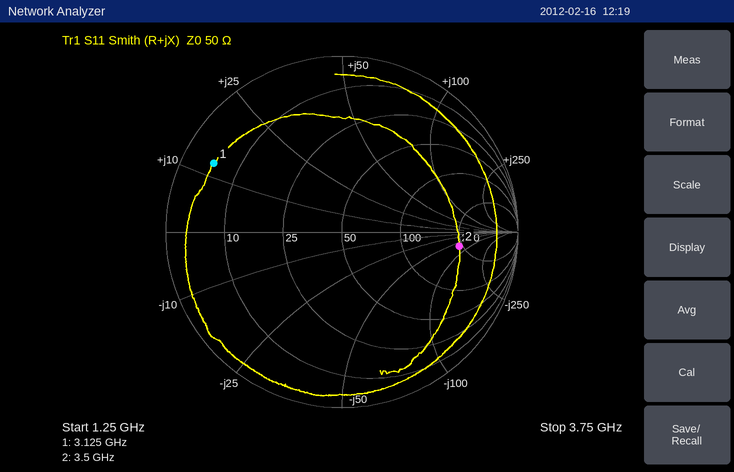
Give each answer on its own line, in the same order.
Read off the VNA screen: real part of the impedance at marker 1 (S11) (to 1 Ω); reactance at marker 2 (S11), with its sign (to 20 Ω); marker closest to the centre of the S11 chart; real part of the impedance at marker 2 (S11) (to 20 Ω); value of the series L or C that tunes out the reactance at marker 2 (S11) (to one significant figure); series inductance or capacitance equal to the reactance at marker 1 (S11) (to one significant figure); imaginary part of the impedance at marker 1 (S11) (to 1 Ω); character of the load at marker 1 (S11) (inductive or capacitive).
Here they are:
5 Ω
-60 Ω
marker 2
240 Ω
3 nH
600 pH
+12 Ω
inductive
